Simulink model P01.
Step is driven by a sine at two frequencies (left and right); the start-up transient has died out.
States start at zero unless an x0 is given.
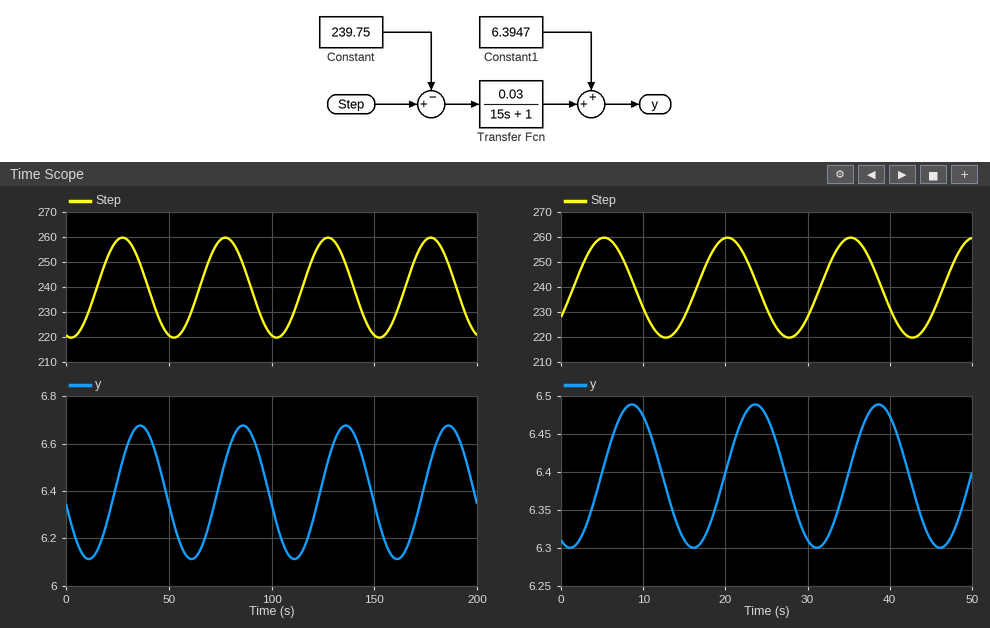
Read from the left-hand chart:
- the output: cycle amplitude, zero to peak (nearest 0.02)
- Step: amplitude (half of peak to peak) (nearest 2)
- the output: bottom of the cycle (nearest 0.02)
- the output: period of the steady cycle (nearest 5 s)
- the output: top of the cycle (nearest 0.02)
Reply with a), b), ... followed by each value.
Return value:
a) 0.28
b) 20
c) 6.12
d) 50 s
e) 6.68
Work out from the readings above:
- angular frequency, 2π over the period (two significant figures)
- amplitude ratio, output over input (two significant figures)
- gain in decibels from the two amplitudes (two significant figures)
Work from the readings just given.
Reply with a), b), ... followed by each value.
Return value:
a) 0.13 rad/s
b) 0.014
c) -37 dB
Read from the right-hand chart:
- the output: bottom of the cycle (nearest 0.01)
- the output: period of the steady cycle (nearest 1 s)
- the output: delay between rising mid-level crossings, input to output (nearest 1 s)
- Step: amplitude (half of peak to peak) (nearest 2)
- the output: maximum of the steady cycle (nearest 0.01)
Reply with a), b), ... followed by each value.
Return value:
a) 6.30
b) 15 s
c) 3 s
d) 20
e) 6.49
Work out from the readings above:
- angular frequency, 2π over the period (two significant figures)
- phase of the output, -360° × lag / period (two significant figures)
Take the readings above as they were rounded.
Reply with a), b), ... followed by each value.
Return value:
a) 0.42 rad/s
b) -72°
